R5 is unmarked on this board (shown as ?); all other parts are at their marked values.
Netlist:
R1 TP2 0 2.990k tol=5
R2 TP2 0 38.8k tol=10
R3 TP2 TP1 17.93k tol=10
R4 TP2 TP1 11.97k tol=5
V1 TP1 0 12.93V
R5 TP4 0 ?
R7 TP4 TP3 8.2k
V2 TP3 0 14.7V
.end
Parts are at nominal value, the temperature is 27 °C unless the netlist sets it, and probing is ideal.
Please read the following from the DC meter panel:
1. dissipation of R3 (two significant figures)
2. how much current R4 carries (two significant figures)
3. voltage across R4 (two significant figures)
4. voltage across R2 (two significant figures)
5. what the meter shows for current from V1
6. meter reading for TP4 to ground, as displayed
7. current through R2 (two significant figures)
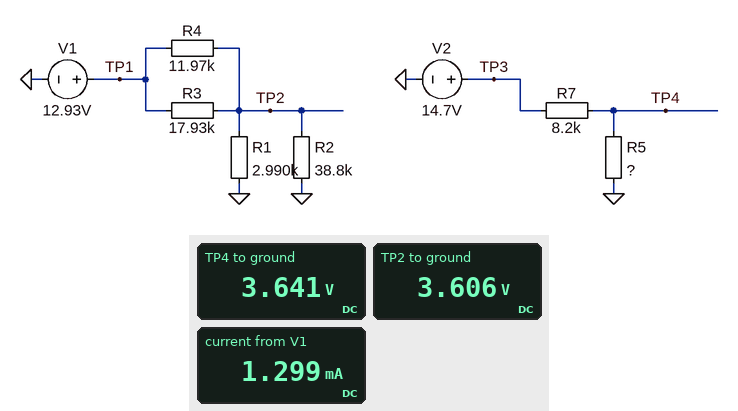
4.8 mW
780 µA
9.3 V
3.6 V
1.299 mA
3.641 V
93 µA
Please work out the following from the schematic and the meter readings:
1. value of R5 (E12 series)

2.7 kΩ
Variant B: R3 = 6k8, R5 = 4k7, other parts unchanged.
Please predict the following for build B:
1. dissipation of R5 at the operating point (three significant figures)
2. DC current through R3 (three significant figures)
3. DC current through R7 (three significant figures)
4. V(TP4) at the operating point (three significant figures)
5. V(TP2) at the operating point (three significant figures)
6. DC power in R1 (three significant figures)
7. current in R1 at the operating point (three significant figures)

6.10 mW
1.16 mA
1.14 mA
5.36 V
5.05 V
8.52 mW
1.69 mA
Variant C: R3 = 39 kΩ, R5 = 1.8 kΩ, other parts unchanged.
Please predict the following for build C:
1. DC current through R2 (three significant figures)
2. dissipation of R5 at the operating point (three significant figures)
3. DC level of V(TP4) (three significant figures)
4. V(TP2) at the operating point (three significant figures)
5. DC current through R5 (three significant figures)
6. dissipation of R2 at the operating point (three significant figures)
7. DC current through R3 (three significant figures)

77.5 µA
3.89 mW
2.65 V
3.01 V
1.47 mA
233 µW
254 µA
